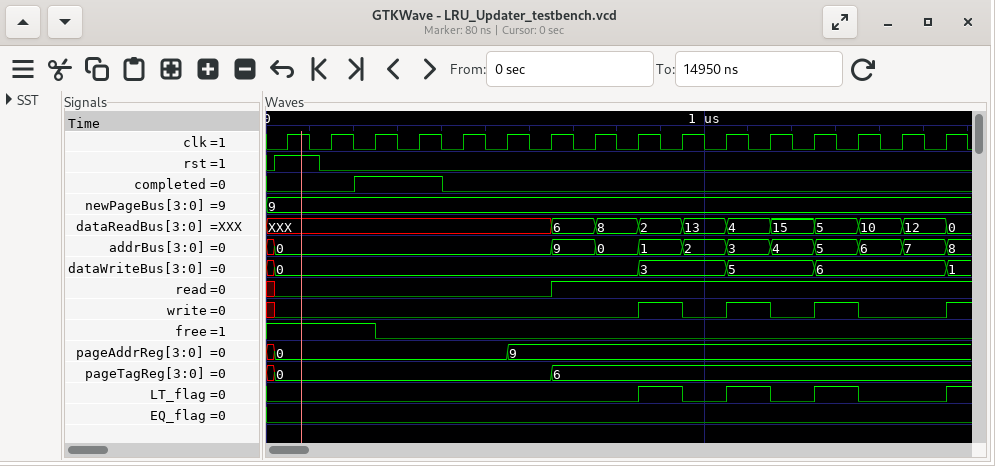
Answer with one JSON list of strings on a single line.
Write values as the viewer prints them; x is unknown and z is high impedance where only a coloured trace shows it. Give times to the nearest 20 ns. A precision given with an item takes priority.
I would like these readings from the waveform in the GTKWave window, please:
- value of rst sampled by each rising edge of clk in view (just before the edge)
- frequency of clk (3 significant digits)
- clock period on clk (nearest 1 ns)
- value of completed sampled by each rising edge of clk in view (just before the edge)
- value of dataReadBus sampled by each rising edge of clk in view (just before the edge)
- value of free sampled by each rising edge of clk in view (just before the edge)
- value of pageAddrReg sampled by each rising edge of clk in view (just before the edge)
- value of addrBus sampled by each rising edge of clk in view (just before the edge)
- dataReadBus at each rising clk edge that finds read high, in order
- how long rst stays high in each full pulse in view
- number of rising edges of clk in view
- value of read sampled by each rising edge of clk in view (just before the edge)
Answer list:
["1 0 0 0 0 0 0 0 0 0 0 0 0 0 0 0", "10.0 MHz", "100 ns", "0 0 1 1 0 0 0 0 0 0 0 0 0 0 0 0", "XXX, XXX, XXX, XXX, XXX, XXX, XXX, 6, 8, 2, 13, 4, 15, 5, 10, 12", "1 1 1 0 0 0 0 0 0 0 0 0 0 0 0 0", "0, 0, 0, 0, 0, 0, 9, 9, 9, 9, 9, 9, 9, 9, 9, 9", "0, 0, 0, 0, 0, 0, 0, 9, 0, 1, 2, 3, 4, 5, 6, 7", "6, 8, 2, 13, 4, 15, 5, 10, 12", "100 ns", "16", "0 0 0 0 0 0 0 1 1 1 1 1 1 1 1 1"]
